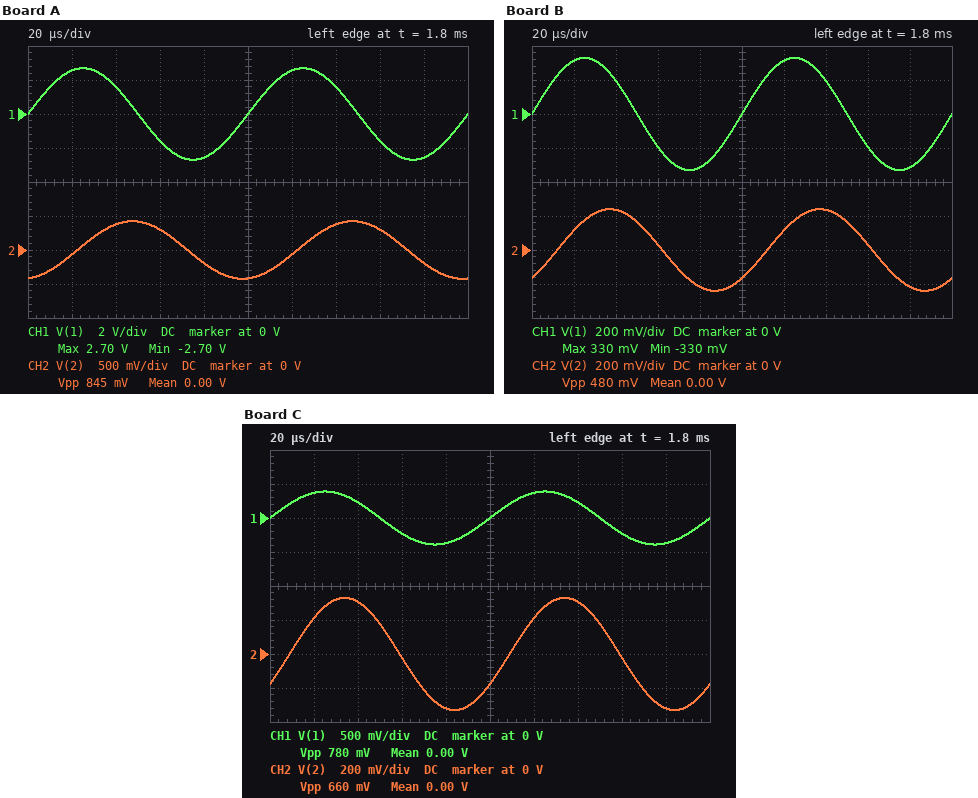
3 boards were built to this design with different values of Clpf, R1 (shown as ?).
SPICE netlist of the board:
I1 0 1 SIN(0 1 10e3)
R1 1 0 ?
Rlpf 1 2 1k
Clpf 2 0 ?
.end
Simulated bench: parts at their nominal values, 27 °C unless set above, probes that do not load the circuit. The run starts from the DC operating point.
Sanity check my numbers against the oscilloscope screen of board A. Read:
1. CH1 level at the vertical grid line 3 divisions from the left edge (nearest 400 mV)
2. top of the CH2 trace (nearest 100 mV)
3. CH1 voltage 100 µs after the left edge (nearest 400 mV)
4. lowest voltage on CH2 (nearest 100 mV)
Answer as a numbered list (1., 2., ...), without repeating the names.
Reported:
1. -1.6 V
2. 400 mV
3. 0 V
4. -400 mV
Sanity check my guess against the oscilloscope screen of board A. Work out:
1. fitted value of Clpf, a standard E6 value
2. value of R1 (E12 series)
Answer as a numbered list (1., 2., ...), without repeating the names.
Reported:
1. 100 nF
2. 2.7 Ω
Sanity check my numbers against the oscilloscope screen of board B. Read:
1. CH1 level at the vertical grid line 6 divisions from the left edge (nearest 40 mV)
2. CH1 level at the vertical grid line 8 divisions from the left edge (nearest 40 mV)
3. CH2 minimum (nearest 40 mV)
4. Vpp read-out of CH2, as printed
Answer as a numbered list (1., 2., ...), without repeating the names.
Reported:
1. 320 mV
2. -200 mV
3. -240 mV
4. 480 mV
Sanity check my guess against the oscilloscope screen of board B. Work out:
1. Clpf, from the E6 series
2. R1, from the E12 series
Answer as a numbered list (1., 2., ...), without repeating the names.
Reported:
1. 15 nF
2. 0.33 Ω
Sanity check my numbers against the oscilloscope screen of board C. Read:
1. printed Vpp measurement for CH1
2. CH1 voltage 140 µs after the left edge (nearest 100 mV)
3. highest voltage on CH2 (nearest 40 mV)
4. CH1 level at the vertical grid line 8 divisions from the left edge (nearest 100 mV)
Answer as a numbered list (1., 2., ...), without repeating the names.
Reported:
1. 780 mV
2. 200 mV
3. 320 mV
4. -200 mV
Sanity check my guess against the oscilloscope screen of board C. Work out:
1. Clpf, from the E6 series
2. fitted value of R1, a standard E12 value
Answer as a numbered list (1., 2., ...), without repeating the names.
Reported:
1. 10 nF
2. 0.39 Ω
